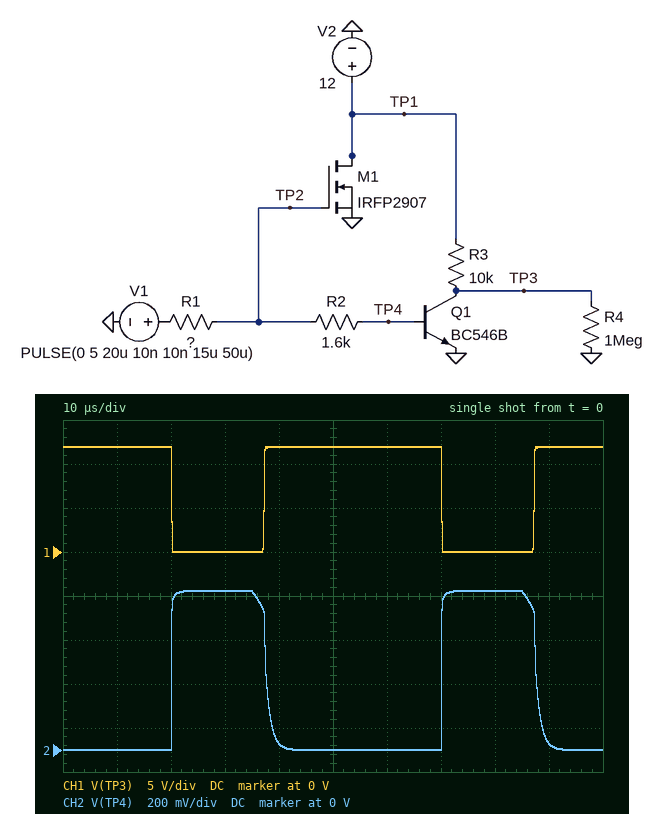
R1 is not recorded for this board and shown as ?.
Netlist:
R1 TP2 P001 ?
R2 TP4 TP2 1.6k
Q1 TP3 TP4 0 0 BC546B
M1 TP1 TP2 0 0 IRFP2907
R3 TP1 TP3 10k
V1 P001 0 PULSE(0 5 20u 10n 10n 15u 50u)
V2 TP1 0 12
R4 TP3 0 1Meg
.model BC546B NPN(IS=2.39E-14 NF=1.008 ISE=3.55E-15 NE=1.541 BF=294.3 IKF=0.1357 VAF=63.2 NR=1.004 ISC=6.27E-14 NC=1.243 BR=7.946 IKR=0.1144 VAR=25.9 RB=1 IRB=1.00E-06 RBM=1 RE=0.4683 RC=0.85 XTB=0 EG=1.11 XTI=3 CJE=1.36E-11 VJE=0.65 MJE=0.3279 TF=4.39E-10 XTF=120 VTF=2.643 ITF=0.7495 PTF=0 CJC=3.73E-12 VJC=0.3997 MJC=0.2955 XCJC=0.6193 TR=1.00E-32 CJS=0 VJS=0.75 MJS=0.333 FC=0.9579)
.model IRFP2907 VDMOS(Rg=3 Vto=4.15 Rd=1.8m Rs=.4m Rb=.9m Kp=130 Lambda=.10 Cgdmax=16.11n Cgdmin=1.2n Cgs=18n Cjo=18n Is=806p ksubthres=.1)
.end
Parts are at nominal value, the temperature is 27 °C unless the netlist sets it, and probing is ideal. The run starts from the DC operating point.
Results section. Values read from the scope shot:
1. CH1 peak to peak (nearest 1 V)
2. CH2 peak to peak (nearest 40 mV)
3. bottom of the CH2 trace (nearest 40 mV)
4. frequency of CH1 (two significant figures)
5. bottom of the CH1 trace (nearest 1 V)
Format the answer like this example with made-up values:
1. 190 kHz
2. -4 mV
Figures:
1. 12 V
2. 720 mV
3. 0 V
4. 20 kHz
5. 0 V
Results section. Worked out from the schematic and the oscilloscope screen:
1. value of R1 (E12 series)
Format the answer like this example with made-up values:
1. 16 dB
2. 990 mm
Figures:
1. 47 Ω
